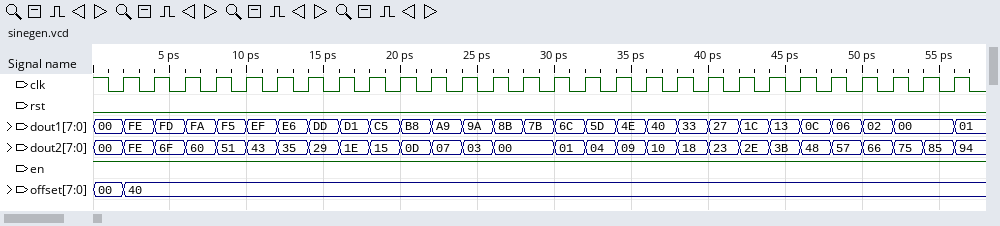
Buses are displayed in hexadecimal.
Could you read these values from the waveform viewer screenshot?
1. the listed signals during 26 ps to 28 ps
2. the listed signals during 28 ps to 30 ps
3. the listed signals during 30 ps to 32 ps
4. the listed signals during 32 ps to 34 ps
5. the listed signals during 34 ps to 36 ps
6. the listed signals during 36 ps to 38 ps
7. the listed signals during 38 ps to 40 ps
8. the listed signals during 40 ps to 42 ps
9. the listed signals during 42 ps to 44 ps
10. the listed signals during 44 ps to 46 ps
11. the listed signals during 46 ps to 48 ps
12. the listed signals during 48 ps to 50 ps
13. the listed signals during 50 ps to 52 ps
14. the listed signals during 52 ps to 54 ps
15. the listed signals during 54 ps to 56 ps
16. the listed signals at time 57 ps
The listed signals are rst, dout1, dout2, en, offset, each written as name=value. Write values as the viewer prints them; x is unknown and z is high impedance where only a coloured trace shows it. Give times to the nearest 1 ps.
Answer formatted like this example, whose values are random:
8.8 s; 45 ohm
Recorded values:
rst=0, dout1=8B, dout2=00, en=1, offset=40; rst=0, dout1=7B, dout2=00, en=1, offset=40; rst=0, dout1=6C, dout2=01, en=1, offset=40; rst=0, dout1=5D, dout2=04, en=1, offset=40; rst=0, dout1=4E, dout2=09, en=1, offset=40; rst=0, dout1=40, dout2=10, en=1, offset=40; rst=0, dout1=33, dout2=18, en=1, offset=40; rst=0, dout1=27, dout2=23, en=1, offset=40; rst=0, dout1=1C, dout2=2E, en=1, offset=40; rst=0, dout1=13, dout2=3B, en=1, offset=40; rst=0, dout1=0C, dout2=48, en=1, offset=40; rst=0, dout1=06, dout2=57, en=1, offset=40; rst=0, dout1=02, dout2=66, en=1, offset=40; rst=0, dout1=00, dout2=75, en=1, offset=40; rst=0, dout1=00, dout2=85, en=1, offset=40; rst=0, dout1=01, dout2=94, en=1, offset=40
